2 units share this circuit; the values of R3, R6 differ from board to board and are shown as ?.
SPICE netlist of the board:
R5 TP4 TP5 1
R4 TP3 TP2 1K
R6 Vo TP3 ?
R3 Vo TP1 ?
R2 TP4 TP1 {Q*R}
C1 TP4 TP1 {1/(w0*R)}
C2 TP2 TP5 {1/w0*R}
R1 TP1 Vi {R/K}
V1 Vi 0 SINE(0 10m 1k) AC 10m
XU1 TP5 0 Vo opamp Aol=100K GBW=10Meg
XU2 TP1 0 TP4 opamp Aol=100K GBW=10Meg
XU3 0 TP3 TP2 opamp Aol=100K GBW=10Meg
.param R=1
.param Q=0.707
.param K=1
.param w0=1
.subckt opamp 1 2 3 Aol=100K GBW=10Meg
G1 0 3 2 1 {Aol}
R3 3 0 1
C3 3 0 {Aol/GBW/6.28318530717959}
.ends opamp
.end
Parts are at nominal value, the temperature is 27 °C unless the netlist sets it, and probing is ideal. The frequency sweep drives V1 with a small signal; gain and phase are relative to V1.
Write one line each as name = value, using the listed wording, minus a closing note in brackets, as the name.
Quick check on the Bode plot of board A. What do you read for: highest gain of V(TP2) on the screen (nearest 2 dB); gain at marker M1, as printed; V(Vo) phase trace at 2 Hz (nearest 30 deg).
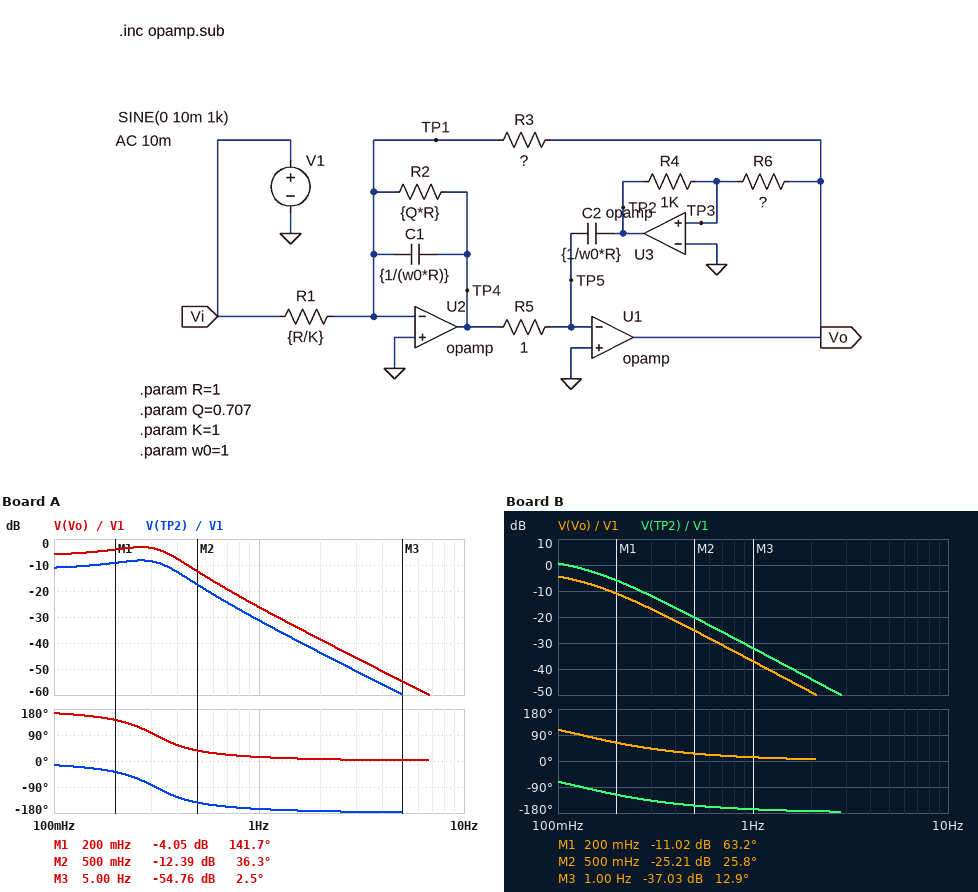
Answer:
highest gain of V(TP2) on the screen = -8 dB
gain at marker M1, as printed = -4.05 dB
V(Vo) phase trace at 2 Hz = 0 deg
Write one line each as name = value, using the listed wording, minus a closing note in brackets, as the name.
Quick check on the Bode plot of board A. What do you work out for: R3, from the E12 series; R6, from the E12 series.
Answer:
R3, from the E12 series = 0.47 Ω
R6, from the E12 series = 1.8 kΩ
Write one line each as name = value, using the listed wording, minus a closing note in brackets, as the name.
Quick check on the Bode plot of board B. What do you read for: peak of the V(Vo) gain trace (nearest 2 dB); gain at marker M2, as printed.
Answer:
peak of the V(Vo) gain trace = -4 dB
gain at marker M2, as printed = -25.21 dB
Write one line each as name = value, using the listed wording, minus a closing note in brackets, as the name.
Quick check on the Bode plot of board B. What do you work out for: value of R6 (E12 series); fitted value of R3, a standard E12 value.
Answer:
value of R6 = 560 Ω
fitted value of R3, a standard E12 value = 0.82 Ω
